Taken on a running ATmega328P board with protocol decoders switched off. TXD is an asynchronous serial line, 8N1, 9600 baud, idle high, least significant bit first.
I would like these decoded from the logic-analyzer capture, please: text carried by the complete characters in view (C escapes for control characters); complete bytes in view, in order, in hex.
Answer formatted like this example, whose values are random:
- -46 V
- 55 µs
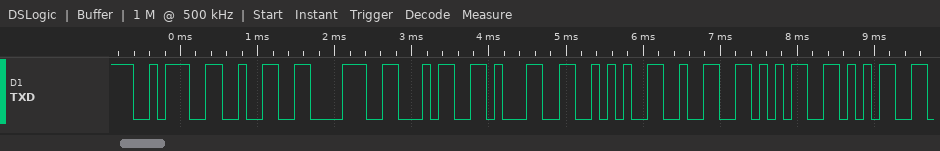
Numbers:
- ":2841*255"
- 0x3A 0x32 0x38 0x34 0x31 0x2A 0x32 0x35 0x35
